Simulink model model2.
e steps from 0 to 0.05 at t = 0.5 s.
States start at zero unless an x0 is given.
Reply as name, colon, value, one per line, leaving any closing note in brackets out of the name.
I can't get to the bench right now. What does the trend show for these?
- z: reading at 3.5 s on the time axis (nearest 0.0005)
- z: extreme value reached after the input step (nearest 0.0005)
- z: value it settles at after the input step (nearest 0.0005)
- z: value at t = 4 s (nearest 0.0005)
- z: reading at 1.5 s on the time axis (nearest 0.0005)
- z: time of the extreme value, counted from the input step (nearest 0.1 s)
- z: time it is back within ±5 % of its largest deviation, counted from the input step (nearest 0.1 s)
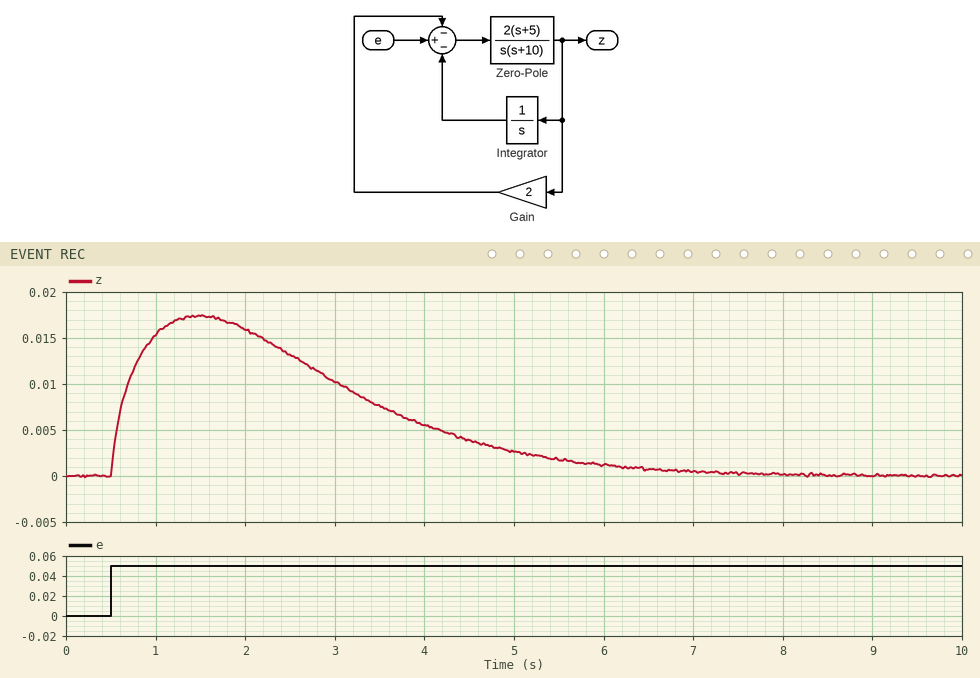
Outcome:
z: reading at 3.5 s on the time axis: 0.0075
z: extreme value reached after the input step: 0.0175
z: value it settles at after the input step: 0.0000
z: value at t = 4 s: 0.0055
z: reading at 1.5 s on the time axis: 0.0175
z: time of the extreme value, counted from the input step: 1.0 s
z: time it is back within ±5 % of its largest deviation, counted from the input step: 5.9 s
